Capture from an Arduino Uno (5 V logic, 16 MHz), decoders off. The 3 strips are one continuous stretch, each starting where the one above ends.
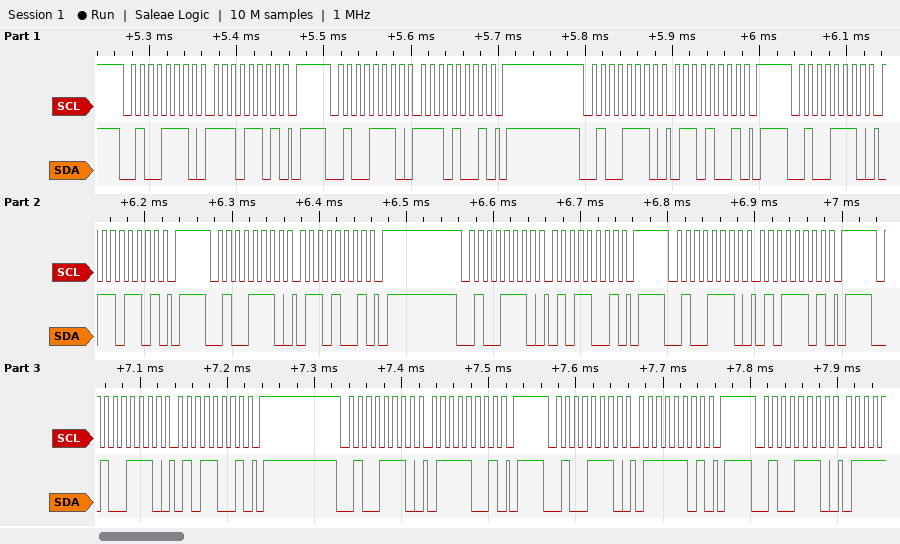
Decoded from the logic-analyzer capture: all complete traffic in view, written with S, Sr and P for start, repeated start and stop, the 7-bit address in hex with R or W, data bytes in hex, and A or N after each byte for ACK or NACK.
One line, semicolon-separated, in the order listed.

S 27W A ED A P S 27W A E9 A P S 27W A 69 A P S 27W A 6D A P S 27W A 69 A P S 27W A 59 A P S 27W A 5D A P S 27W A 59 A P S 27W A 79 A P S 27W A 7D A P S 27W A
